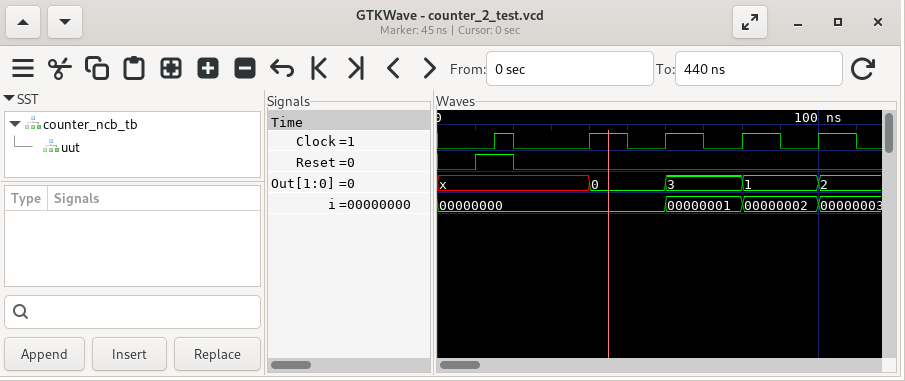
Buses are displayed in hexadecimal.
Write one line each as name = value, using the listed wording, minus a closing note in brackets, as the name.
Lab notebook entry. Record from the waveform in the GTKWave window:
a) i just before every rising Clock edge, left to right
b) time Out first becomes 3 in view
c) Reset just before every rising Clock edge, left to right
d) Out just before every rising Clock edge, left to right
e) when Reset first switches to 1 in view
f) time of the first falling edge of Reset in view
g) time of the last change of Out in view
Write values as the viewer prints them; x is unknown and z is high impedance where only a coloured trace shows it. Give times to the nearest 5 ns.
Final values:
i just before every rising Clock edge, left to right = 00000000, 00000000, 00000000, 00000001, 00000002
time Out first becomes 3 in view = 60 ns
Reset just before every rising Clock edge, left to right = 1 0 0 0 0
Out just before every rising Clock edge, left to right = x, x, 0, 3, 1
when Reset first switches to 1 in view = 10 ns
time of the first falling edge of Reset in view = 20 ns
time of the last change of Out in view = 100 ns
